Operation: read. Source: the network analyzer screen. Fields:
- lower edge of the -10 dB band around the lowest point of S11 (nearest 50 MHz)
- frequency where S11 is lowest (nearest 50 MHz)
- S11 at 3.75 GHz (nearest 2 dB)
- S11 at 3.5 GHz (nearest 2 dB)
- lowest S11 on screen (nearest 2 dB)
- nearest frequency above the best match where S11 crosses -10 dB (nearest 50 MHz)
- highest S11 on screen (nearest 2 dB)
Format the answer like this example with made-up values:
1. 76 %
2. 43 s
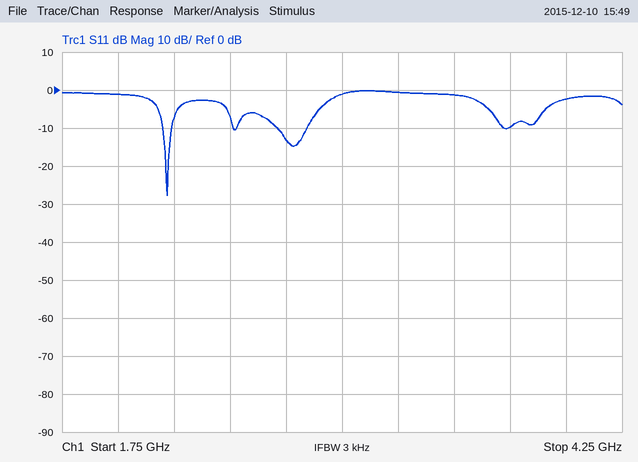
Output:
1. 2.20 GHz
2. 2.20 GHz
3. -10 dB
4. -2 dB
5. -28 dB
6. 2.25 GHz
7. 0 dB
